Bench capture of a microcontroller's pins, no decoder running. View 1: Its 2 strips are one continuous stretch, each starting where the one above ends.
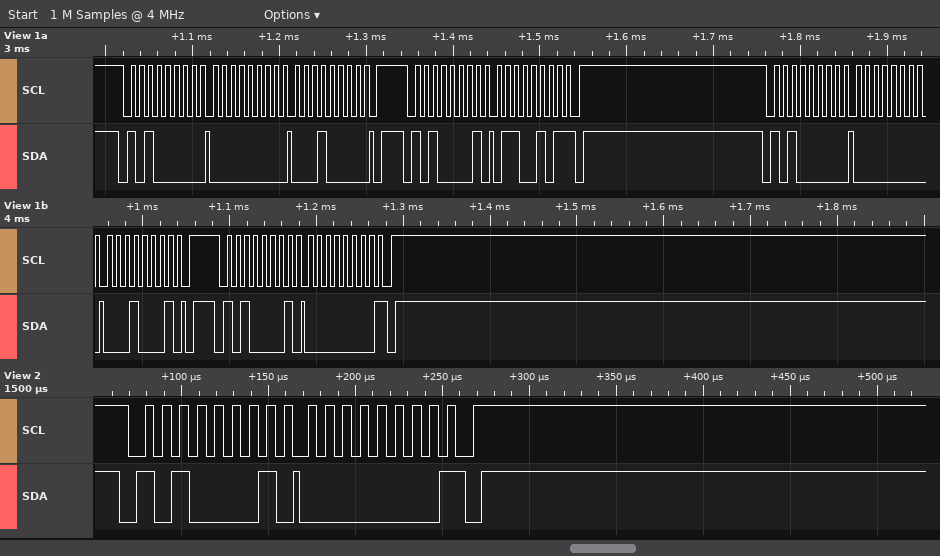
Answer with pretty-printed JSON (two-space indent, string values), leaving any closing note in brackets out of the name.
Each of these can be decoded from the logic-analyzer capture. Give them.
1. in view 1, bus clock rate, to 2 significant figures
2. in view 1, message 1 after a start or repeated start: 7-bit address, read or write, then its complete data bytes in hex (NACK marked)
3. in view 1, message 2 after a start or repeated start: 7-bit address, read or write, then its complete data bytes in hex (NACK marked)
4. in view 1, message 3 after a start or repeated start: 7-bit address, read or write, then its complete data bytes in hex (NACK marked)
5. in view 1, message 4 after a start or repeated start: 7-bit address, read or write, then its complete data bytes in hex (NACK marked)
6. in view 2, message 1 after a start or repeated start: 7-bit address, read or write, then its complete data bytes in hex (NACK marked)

{
  "in view 1, bus clock rate, to 2 significant figures": "100 kHz",
  "in view 1, message 1 after a start or repeated start: 7-bit address, read or write, then its complete data bytes in hex": "0x50 write: 00 10",
  "in view 1, message 2 after a start or repeated start: 7-bit address, read or write, then its complete data bytes in hex": "0x50 read: 65 NACK",
  "in view 1, message 3 after a start or repeated start: 7-bit address, read or write, then its complete data bytes in hex": "0x50 write: 00 11",
  "in view 1, message 4 after a start or repeated start: 7-bit address, read or write, then its complete data bytes in hex": "0x50 read: 00 NACK",
  "in view 2, message 1 after a start or repeated start: 7-bit address, read or write, then its complete data bytes in hex": "0x50 read: 00 NACK"
}
